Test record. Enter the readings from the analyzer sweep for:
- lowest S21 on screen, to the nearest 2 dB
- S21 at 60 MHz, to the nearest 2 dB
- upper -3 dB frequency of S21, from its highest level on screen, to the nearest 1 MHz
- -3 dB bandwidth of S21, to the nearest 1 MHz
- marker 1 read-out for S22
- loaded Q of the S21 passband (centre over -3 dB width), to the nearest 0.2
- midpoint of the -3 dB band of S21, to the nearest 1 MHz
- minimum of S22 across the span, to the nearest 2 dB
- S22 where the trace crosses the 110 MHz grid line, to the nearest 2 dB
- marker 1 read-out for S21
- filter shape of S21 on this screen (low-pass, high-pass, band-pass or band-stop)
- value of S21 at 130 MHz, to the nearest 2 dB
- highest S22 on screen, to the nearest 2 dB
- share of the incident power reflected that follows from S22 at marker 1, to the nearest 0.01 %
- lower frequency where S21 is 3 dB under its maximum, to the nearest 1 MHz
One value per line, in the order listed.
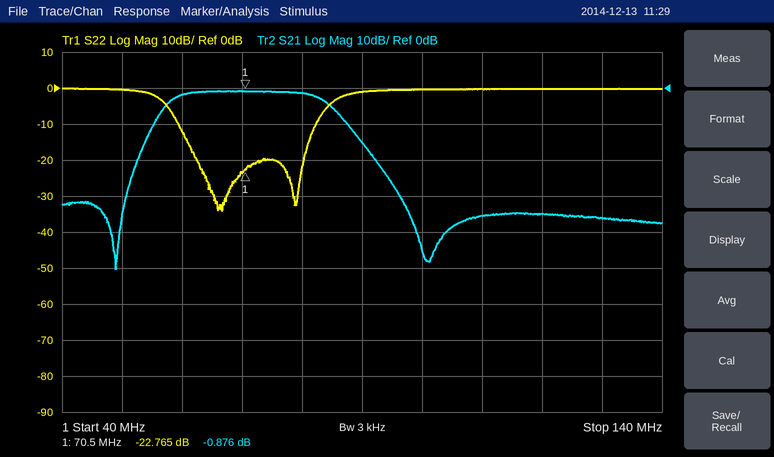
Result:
-50 dB
-2 dB
84 MHz
26 MHz
-22.765 dB
2.8
71 MHz
-34 dB
0 dB
-0.876 dB
band-pass
-36 dB
0 dB
0.53 %
58 MHz
